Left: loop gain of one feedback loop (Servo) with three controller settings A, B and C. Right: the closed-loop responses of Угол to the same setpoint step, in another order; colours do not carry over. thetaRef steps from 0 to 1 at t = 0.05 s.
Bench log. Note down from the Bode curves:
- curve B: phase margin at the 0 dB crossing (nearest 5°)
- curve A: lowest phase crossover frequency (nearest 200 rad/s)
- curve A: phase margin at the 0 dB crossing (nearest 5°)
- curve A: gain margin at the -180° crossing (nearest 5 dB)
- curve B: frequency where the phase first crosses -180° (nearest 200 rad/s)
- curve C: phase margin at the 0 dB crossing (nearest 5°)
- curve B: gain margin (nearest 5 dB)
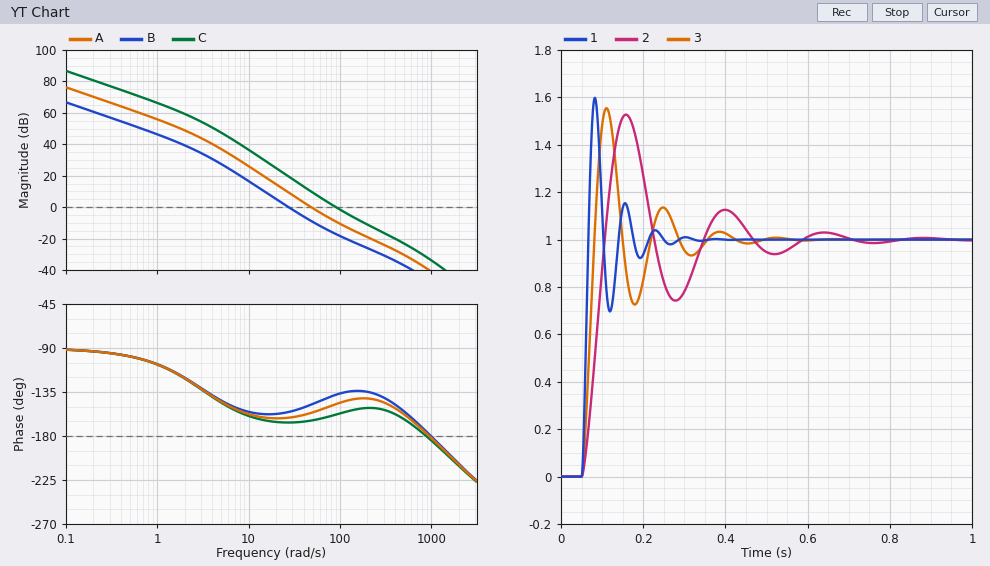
25°
1000 rad/s
25°
40 dB
1000 rad/s
20°
40 dB
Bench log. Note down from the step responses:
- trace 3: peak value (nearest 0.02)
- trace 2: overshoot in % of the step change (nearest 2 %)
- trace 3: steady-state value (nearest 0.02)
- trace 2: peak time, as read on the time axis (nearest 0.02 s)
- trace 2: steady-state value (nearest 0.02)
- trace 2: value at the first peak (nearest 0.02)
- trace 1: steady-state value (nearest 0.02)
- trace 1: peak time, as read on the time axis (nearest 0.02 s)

1.56
52 %
1.00
0.16 s
1.00
1.52
1.00
0.08 s
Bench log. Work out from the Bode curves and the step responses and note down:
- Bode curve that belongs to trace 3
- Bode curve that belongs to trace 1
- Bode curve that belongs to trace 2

A
C
B
